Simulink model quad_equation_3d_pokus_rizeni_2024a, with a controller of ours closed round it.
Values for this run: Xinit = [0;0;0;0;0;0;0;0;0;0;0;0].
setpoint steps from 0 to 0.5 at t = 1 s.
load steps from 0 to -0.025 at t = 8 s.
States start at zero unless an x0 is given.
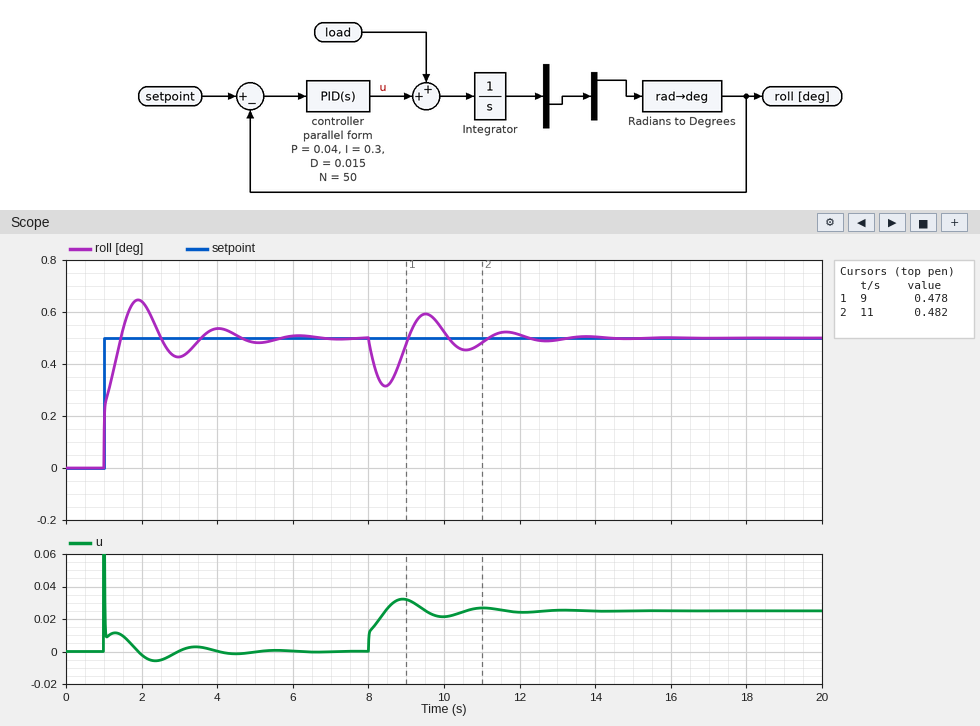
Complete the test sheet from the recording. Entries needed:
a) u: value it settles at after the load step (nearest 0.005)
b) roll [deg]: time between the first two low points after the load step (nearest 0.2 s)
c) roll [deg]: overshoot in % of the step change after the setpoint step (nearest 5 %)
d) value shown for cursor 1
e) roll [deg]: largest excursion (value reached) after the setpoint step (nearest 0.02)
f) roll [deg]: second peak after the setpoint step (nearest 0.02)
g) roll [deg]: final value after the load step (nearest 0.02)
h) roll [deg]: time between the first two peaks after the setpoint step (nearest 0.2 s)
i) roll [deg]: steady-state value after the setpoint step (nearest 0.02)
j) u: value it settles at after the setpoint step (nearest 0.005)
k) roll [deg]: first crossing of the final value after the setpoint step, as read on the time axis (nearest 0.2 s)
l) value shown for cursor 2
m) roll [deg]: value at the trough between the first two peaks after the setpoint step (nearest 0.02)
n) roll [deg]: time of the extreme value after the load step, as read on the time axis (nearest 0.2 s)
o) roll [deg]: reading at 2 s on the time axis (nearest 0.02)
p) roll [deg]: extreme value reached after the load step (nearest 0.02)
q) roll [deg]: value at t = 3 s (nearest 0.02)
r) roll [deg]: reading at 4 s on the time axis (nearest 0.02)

0.025
2.2 s
30 %
0.478
0.64
0.54
0.50
2.2 s
0.50
0.000
1.4 s
0.482
0.42
8.4 s
0.64
0.32
0.42
0.54
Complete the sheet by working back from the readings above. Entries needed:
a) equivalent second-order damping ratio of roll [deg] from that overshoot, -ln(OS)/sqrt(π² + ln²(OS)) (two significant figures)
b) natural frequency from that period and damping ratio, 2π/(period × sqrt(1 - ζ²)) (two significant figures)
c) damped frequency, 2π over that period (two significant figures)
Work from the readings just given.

0.36
3.1 rad/s
2.9 rad/s
